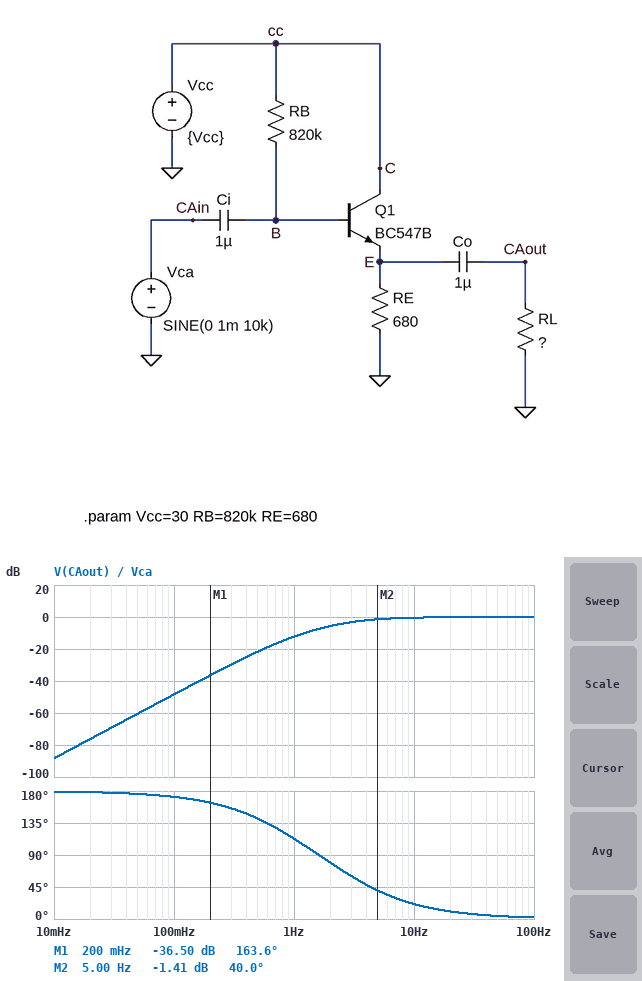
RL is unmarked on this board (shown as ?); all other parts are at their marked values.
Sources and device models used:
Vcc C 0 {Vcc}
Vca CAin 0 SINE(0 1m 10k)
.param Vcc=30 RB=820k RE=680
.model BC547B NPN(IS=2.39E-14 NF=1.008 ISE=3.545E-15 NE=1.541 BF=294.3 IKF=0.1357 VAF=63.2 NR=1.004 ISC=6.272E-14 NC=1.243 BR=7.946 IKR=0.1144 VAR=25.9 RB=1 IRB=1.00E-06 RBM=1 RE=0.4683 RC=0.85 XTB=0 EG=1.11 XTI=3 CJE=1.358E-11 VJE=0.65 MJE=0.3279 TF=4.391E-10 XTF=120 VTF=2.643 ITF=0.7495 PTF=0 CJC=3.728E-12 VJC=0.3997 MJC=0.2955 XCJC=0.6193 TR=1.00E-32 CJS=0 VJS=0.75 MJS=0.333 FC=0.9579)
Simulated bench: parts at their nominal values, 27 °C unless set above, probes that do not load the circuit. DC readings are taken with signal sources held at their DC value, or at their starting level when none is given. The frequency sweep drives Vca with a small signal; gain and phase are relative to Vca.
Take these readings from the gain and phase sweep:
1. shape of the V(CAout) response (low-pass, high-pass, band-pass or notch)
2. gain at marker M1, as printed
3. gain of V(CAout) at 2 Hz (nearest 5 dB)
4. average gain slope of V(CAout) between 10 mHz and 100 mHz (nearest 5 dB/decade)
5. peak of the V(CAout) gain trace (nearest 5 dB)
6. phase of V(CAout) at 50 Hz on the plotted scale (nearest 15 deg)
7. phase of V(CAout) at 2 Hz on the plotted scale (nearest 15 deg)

high-pass
-36.50 dB
-5 dB
40 dB/decade
0 dB
0 deg
75 deg
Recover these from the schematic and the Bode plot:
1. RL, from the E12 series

56 kΩ
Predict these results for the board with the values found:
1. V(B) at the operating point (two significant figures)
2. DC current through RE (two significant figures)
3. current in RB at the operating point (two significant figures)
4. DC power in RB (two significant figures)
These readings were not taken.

7.6 V
10 mA
27 µA
610 µW
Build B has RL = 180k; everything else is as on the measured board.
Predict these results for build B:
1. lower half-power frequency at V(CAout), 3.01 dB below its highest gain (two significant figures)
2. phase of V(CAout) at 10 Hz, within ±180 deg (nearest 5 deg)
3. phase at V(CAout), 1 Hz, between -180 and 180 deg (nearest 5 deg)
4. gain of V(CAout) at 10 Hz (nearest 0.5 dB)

1.4 Hz
10 deg
85 deg
0 dB
